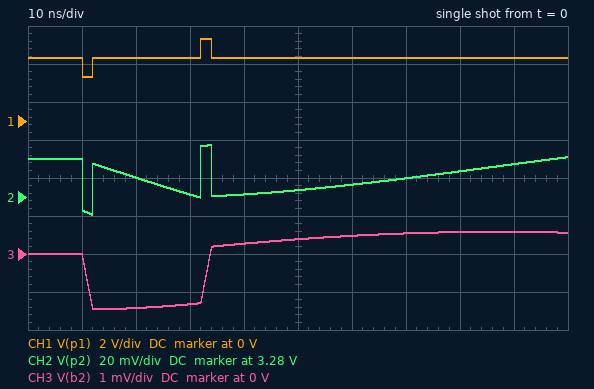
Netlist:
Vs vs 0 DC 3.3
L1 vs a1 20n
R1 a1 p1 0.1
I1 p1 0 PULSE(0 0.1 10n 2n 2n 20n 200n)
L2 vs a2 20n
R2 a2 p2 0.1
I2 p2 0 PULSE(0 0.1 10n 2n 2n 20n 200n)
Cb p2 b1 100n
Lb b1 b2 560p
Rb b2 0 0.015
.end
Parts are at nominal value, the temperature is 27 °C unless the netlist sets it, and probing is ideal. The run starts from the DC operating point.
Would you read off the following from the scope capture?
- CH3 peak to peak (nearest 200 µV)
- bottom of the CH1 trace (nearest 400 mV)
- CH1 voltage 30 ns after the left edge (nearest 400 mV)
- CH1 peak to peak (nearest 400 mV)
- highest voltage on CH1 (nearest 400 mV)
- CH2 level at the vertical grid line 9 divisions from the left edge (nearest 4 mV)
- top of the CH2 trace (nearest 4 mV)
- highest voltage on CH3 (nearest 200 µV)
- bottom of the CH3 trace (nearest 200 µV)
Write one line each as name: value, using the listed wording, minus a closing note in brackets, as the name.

CH3 peak to peak: 2.0 mV
bottom of the CH1 trace: 2.4 V
CH1 voltage 30 ns after the left edge: 3.2 V
CH1 peak to peak: 2.0 V
highest voltage on CH1: 4.4 V
CH2 level at the vertical grid line 9 divisions from the left edge: 3.296 V
top of the CH2 trace: 3.308 V
highest voltage on CH3: 600 µV
bottom of the CH3 trace: -1.4 mV
